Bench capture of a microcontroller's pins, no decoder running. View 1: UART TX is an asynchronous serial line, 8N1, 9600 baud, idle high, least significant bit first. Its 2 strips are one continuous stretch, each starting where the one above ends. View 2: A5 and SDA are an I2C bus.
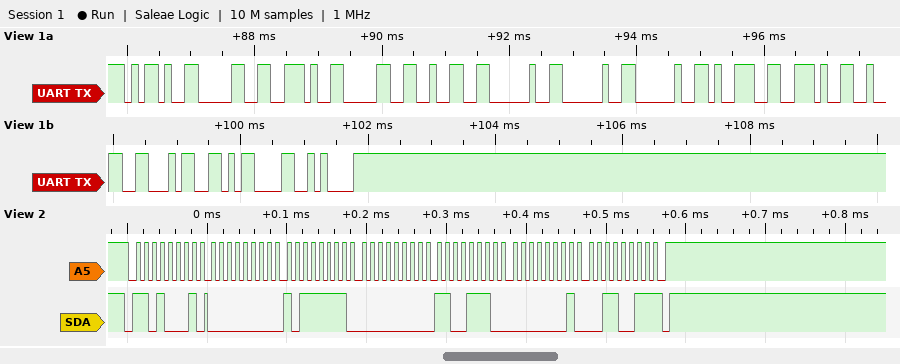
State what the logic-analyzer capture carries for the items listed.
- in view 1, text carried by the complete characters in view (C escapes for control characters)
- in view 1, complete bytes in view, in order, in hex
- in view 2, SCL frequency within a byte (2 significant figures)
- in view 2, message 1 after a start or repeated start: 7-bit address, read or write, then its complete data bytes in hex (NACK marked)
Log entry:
"-0.02   9.24\r\n"
2D 30 2E 30 32 20 20 20 39 2E 32 34 0D 0A
100 kHz
0x68 read: 00 BF 00 CE 01 33 NACK
